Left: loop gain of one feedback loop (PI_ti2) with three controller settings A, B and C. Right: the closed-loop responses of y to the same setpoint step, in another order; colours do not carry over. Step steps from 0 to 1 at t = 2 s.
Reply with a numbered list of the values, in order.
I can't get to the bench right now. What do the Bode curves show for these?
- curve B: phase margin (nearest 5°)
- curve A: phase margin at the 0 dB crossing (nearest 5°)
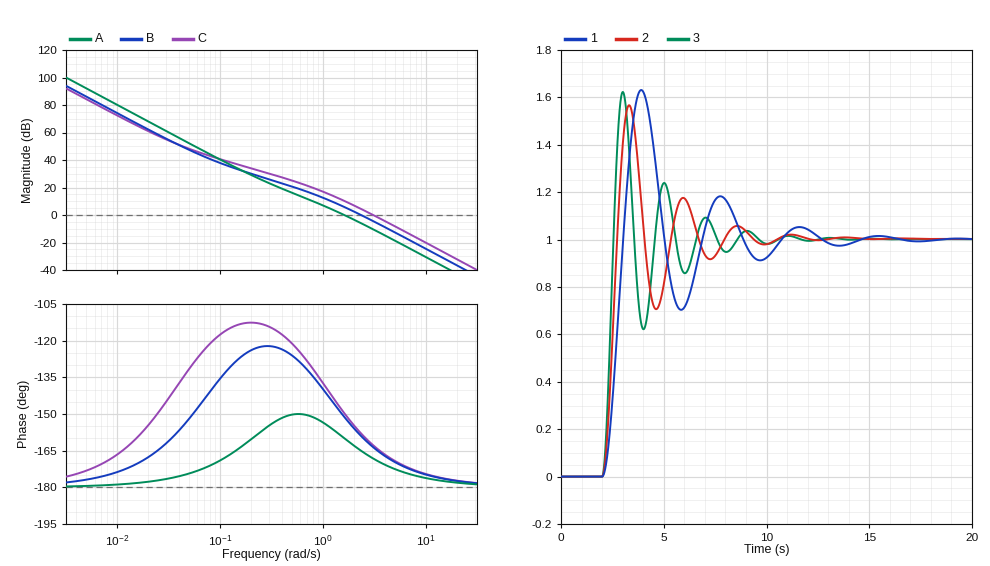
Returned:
1. 20°
2. 20°
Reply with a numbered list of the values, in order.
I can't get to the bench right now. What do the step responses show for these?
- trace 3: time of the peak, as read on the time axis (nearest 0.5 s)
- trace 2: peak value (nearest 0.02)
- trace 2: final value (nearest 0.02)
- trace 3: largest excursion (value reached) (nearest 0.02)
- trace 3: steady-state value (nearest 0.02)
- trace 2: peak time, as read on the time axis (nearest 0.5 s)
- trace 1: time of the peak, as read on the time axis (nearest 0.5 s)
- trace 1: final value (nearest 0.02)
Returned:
1. 3.0 s
2. 1.56
3. 1.00
4. 1.62
5. 1.00
6. 3.5 s
7. 4.0 s
8. 1.00
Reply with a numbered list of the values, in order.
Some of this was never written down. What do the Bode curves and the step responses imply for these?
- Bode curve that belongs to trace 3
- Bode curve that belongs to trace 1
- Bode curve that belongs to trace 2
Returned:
1. C
2. A
3. B
